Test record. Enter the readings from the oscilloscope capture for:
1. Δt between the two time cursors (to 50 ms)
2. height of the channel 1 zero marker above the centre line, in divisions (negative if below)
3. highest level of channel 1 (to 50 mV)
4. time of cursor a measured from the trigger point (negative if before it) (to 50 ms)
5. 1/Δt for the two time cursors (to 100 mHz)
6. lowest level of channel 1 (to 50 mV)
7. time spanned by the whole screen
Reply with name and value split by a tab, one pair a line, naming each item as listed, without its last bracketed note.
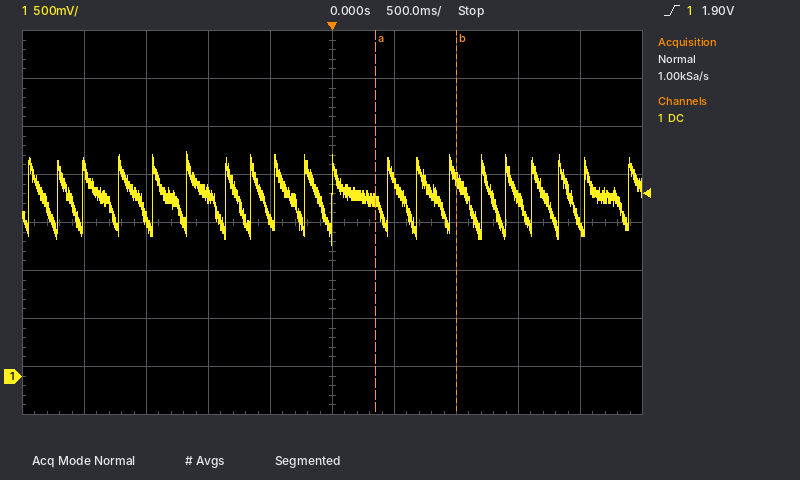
Δt between the two time cursors	650 ms
height of the channel 1 zero marker above the centre line, in divisions	-3.2 div
highest level of channel 1	2.35 V
time of cursor a measured from the trigger point (negative if before it)	+350 ms
1/Δt for the two time cursors	1.5 Hz
lowest level of channel 1	1.35 V
time spanned by the whole screen	5 s
